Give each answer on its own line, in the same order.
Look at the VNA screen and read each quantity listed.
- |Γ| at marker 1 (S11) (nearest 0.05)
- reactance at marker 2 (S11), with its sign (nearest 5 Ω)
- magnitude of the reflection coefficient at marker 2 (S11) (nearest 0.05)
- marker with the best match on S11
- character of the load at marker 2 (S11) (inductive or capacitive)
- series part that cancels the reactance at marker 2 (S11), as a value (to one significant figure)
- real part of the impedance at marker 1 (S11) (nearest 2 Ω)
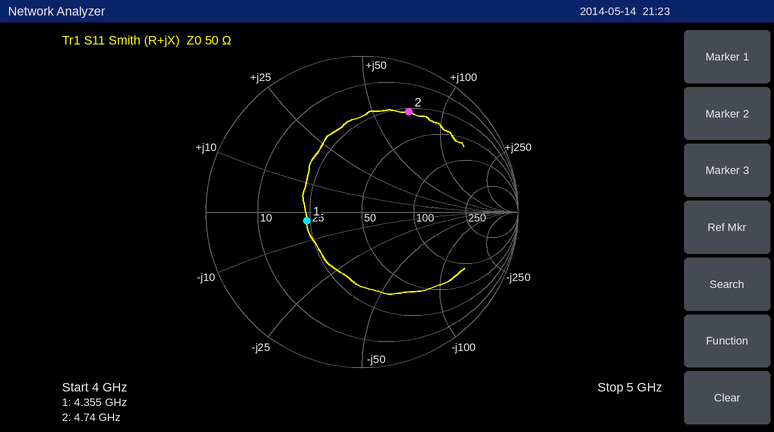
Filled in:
0.35
+70 Ω
0.70
marker 1
inductive
500 fF
24 Ω
